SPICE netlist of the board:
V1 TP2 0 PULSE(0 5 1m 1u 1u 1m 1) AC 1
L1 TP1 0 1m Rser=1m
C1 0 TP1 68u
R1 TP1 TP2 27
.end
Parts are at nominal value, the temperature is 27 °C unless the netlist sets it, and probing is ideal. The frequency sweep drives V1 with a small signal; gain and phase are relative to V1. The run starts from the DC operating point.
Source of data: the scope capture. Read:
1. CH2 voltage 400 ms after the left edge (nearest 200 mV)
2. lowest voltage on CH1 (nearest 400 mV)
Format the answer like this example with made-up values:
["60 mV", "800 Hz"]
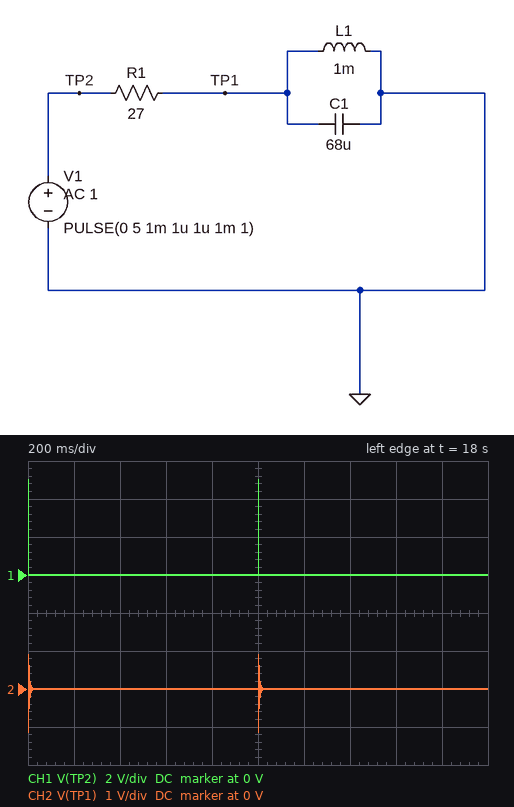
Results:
["0 V", "0 V"]
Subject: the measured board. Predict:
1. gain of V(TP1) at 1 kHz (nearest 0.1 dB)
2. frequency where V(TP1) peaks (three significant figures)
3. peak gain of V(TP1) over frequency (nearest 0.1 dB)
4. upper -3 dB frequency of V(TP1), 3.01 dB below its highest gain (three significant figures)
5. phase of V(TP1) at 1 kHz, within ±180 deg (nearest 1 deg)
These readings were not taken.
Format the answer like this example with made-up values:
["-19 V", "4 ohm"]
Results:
["-17.3 dB", "610 Hz", "0 dB", "655 Hz", "-82 deg"]
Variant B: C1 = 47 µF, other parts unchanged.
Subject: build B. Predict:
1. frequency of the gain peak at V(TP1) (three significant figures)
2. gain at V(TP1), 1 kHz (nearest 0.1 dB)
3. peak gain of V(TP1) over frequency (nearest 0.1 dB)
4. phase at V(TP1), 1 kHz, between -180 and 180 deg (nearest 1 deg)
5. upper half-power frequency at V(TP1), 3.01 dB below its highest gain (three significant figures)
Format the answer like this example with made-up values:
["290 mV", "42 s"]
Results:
["734 Hz", "-11.6 dB", "0 dB", "-75 deg", "800 Hz"]
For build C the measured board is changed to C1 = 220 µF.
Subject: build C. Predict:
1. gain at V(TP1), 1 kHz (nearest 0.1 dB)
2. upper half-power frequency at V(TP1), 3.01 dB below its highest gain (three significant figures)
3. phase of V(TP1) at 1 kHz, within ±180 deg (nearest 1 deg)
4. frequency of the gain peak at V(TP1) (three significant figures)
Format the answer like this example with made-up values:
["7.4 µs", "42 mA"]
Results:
["-30.4 dB", "353 Hz", "-88 deg", "339 Hz"]
